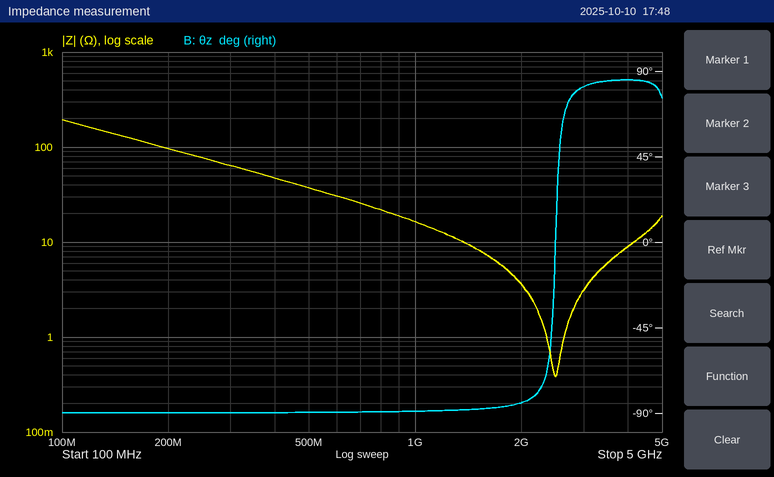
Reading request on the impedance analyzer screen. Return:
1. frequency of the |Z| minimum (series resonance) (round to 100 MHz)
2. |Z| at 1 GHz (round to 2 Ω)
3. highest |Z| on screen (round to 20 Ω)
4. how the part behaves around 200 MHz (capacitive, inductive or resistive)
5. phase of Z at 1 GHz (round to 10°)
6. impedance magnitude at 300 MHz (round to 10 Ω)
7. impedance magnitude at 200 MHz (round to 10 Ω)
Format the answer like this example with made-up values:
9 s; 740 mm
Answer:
2.5 GHz; 16 Ω; 200 Ω; capacitive; -90°; 60 Ω; 100 Ω
